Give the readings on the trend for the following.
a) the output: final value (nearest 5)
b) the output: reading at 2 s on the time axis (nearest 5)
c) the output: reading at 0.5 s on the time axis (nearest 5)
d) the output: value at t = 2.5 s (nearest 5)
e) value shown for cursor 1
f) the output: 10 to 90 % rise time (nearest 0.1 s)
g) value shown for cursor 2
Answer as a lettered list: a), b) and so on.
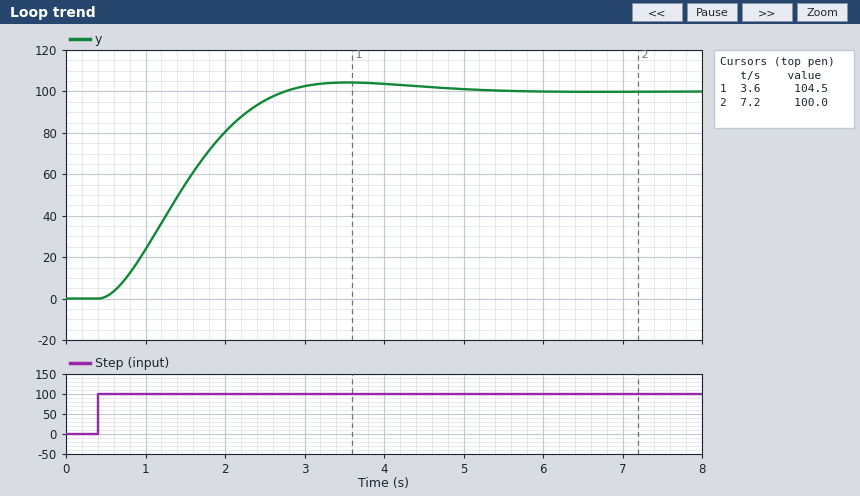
a) 100
b) 80
c) 0
d) 95
e) 104.5
f) 1.5 s
g) 100.0
